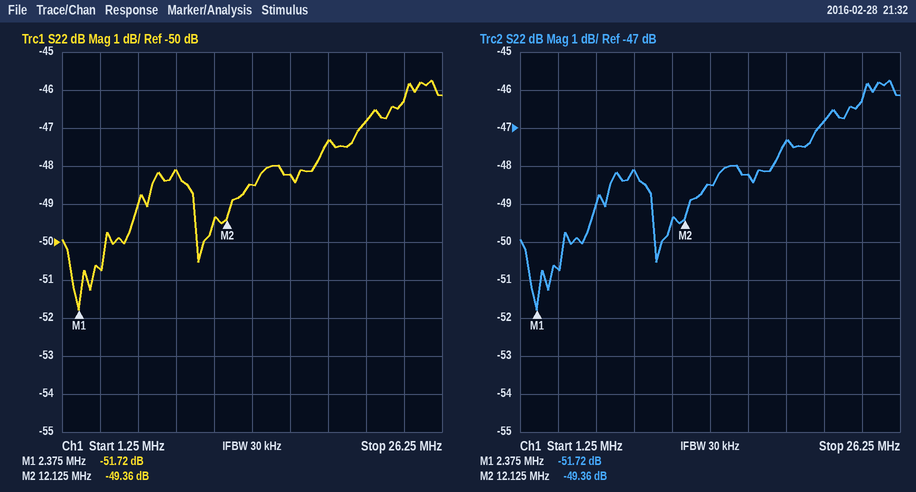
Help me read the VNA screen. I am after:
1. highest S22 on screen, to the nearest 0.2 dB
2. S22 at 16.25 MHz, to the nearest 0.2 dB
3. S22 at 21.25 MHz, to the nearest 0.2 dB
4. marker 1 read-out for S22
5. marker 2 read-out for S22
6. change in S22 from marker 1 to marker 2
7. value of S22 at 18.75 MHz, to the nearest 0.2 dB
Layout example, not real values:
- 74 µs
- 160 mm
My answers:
- -45.8 dB
- -48.2 dB
- -46.8 dB
- -51.72 dB
- -49.36 dB
- 2.36 dB
- -47.4 dB
